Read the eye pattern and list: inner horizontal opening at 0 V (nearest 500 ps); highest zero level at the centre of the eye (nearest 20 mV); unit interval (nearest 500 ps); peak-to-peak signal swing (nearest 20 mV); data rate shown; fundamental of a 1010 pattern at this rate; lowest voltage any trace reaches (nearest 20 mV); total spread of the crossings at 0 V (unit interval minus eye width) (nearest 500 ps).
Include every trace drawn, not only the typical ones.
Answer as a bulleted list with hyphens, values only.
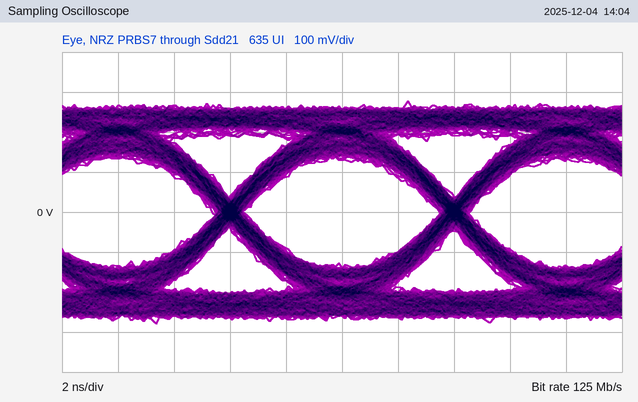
- 7.0 ns
- -140 mV
- 8.0 ns
- 560 mV
- 125 Mb/s
- 62.5 MHz
- -280 mV
- 1.0 ns
